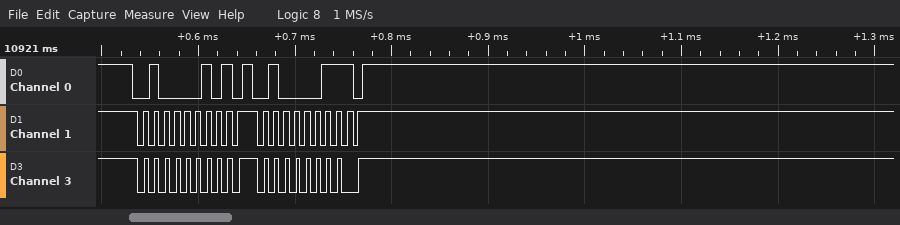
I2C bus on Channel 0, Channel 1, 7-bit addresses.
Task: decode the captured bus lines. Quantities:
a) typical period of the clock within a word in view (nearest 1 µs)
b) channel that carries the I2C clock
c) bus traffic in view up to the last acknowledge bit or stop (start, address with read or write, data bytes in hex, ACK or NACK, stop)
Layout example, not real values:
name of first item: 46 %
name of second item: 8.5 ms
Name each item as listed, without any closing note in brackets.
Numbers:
typical period of the clock within a word in view: 11 µs
channel that carries the I2C clock: Channel 1
bus traffic in view up to the last acknowledge bit or stop: start, address 21 write NACK, stop, start, address 21 read NACK, stop
